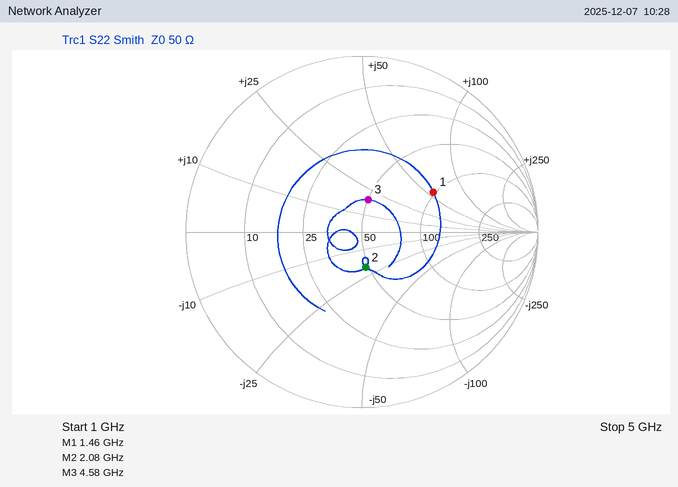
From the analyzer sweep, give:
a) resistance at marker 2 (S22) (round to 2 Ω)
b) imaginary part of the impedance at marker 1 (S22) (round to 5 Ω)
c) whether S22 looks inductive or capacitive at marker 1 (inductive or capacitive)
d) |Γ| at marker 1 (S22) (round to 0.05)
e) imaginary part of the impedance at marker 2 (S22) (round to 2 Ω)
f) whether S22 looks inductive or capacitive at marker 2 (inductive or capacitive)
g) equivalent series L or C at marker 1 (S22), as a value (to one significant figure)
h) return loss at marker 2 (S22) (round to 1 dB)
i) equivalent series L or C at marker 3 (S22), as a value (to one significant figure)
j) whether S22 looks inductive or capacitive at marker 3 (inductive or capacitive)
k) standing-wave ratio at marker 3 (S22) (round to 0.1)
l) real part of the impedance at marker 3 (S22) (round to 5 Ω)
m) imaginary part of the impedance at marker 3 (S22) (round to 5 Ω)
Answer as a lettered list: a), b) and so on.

a) 48 Ω
b) +55 Ω
c) inductive
d) 0.45
e) -20 Ω
f) capacitive
g) 6 nH
h) 14 dB
i) 700 pH
j) inductive
k) 1.5
l) 50 Ω
m) +20 Ω
